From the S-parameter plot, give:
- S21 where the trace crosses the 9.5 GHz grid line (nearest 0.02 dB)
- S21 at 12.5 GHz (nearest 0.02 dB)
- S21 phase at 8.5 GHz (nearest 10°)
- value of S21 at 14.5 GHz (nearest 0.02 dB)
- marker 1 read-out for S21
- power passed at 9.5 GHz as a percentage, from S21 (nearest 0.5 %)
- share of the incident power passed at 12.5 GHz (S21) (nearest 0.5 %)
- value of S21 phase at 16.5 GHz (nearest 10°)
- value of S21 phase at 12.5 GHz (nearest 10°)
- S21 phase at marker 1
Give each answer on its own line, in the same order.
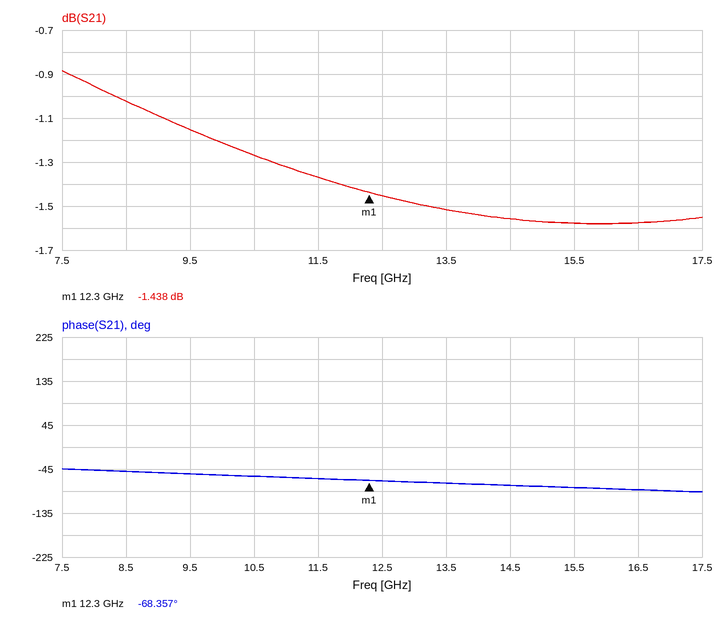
-1.16 dB
-1.46 dB
-50°
-1.56 dB
-1.438 dB
76.5 %
71.5 %
-90°
-70°
-68.357°
